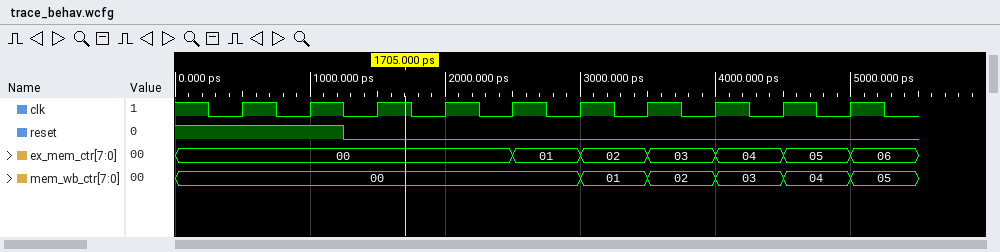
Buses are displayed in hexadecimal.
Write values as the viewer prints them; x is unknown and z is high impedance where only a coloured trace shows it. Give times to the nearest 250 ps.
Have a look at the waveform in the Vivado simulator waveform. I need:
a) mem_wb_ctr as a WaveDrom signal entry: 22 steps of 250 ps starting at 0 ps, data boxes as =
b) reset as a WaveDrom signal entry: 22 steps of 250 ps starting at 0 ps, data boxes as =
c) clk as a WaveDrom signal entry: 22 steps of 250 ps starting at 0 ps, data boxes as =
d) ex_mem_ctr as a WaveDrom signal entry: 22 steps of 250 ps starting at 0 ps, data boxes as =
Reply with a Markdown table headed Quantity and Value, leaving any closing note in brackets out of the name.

| Quantity | Value |
|---|---|
| mem_wb_ctr as a WaveDrom signal entry: 22 steps of 250 ps starting at 0 ps, data boxes as = | {name: 'mem_wb_ctr', wave: '=...........=.=.=.=.=.', data: '00 01 02 03 04 05'} |
| reset as a WaveDrom signal entry: 22 steps of 250 ps starting at 0 ps, data boxes as = | {name: 'reset', wave: '1....0................'} |
| clk as a WaveDrom signal entry: 22 steps of 250 ps starting at 0 ps, data boxes as = | {name: 'clk', wave: '1010101010101010101010'} |
| ex_mem_ctr as a WaveDrom signal entry: 22 steps of 250 ps starting at 0 ps, data boxes as = | {name: 'ex_mem_ctr', wave: '=.........=.=.=.=.=.=.', data: '00 01 02 03 04 05 06'} |
